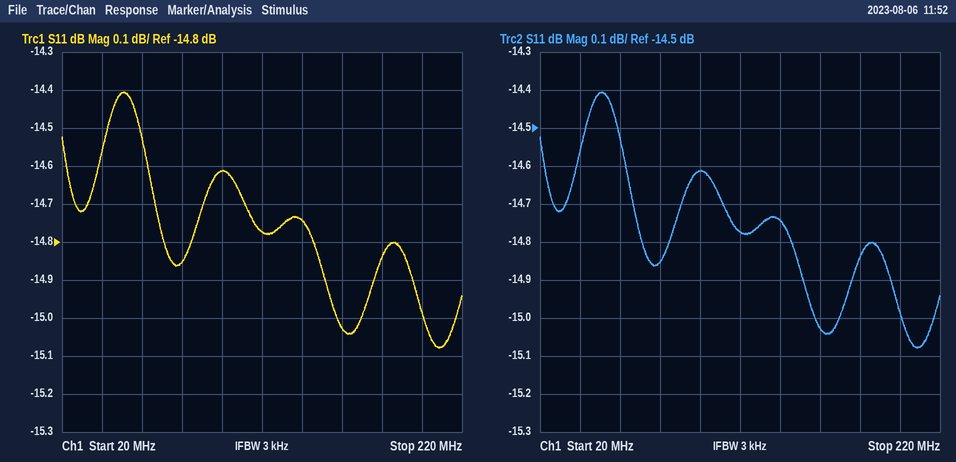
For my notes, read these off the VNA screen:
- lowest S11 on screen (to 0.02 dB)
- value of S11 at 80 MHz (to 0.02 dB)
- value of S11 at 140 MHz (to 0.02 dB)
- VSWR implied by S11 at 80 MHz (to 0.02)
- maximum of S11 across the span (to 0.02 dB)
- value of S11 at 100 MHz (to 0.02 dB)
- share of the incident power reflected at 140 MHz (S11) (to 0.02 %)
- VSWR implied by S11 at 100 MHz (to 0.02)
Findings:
-15.08 dB
-14.86 dB
-14.74 dB
1.44
-14.40 dB
-14.62 dB
3.36 %
1.46
